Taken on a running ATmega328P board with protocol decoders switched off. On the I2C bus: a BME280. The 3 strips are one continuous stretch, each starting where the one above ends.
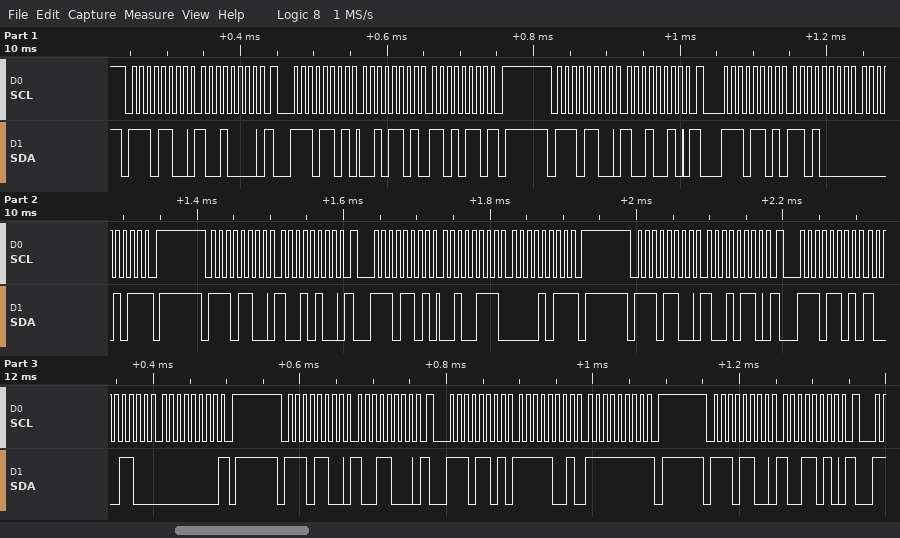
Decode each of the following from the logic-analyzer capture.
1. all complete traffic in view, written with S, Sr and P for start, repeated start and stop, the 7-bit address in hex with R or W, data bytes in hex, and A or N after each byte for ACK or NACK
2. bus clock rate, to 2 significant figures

S 76W A 90 A Sr 76R A 2D A D6 N P S 76W A 92 A Sr 76R A D0 A 0B N P S 76W A 94 A Sr 76R A 27 A 0B N P S 76W A 96 A Sr 76R A 8C A 00 N P S 76W A 98 A Sr 76R A F9 A FF N P S 76W A 9A A
100 kHz
